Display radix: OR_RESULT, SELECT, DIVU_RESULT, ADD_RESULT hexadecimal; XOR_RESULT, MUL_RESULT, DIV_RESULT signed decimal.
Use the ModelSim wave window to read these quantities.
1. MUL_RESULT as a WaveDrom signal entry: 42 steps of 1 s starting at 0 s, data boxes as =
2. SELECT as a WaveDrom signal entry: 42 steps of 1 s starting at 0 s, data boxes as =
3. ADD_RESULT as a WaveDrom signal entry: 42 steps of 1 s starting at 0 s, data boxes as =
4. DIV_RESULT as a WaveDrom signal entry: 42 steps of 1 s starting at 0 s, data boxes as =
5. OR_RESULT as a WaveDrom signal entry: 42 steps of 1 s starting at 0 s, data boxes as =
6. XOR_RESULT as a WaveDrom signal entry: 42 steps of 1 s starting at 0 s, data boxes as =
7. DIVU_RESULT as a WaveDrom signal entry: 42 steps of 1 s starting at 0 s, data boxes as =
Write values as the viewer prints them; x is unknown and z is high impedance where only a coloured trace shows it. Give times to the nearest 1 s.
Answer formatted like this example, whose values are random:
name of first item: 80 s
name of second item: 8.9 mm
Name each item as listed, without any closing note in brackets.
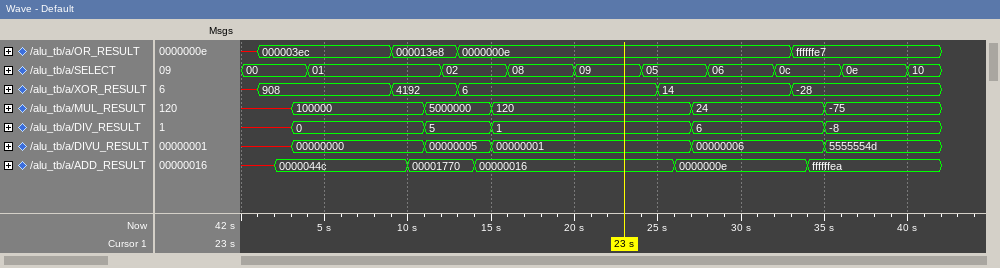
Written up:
MUL_RESULT as a WaveDrom signal entry: 42 steps of 1 s starting at 0 s, data boxes as =: {name: 'MUL_RESULT', wave: 'x..=.......=...=...........=.......=......', data: '100000 5000000 120 24 -75'}
SELECT as a WaveDrom signal entry: 42 steps of 1 s starting at 0 s, data boxes as =: {name: 'SELECT', wave: '=...=.......=...=...=...=...=...=...=...=.', data: '00 01 02 08 09 05 06 0c 0e 10'}
ADD_RESULT as a WaveDrom signal entry: 42 steps of 1 s starting at 0 s, data boxes as =: {name: 'ADD_RESULT', wave: 'x.=.......=...=...........=.......=.......', data: '0000044c 00001770 00000016 0000000e ffffffea'}
DIV_RESULT as a WaveDrom signal entry: 42 steps of 1 s starting at 0 s, data boxes as =: {name: 'DIV_RESULT', wave: 'x..=.......=...=...........=.......=......', data: '0 5 1 6 -8'}
OR_RESULT as a WaveDrom signal entry: 42 steps of 1 s starting at 0 s, data boxes as =: {name: 'OR_RESULT', wave: 'x=.......=...=...................=........', data: '000003ec 000013e8 0000000e ffffffe7'}
XOR_RESULT as a WaveDrom signal entry: 42 steps of 1 s starting at 0 s, data boxes as =: {name: 'XOR_RESULT', wave: 'x=.......=...=...........=.......=........', data: '908 4192 6 14 -28'}
DIVU_RESULT as a WaveDrom signal entry: 42 steps of 1 s starting at 0 s, data boxes as =: {name: 'DIVU_RESULT', wave: 'x..=.......=...=...........=.......=......', data: '00000000 00000005 00000001 00000006 5555554d'}
